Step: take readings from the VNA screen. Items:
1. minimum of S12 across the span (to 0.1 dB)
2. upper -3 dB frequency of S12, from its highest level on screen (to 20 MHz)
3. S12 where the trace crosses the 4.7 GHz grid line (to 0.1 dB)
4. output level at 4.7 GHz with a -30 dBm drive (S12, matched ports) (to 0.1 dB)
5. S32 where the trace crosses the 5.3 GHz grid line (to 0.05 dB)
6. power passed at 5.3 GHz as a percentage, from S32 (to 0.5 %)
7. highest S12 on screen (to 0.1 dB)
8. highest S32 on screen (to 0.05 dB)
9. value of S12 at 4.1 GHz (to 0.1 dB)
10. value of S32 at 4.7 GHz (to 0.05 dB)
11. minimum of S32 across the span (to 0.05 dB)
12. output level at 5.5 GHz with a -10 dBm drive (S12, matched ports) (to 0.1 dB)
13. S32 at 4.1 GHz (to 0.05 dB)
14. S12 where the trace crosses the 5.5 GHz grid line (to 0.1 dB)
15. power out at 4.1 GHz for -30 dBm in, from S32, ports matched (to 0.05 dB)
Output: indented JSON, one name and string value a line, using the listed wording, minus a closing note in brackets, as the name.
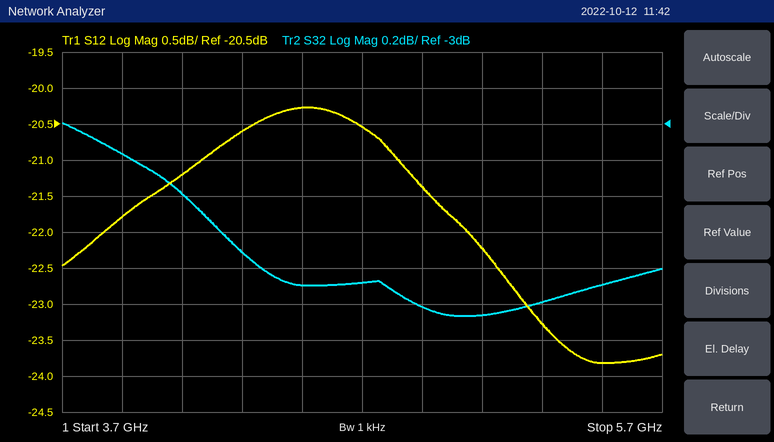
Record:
{
  "minimum of S12 across the span": "-23.8 dB",
  "upper -3 dB frequency of S12, from its highest level on screen": "5.30 GHz",
  "S12 where the trace crosses the 4.7 GHz grid line": "-20.5 dB",
  "output level at 4.7 GHz with a -30 dBm drive (S12, matched ports)": "-50.5 dBm",
  "S32 where the trace crosses the 5.3 GHz grid line": "-4.00 dB",
  "power passed at 5.3 GHz as a percentage, from S32": "40.0 %",
  "highest S12 on screen": "-20.3 dB",
  "highest S32 on screen": "-3.00 dB",
  "value of S12 at 4.1 GHz": "-21.2 dB",
  "value of S32 at 4.7 GHz": "-3.90 dB",
  "minimum of S32 across the span": "-4.05 dB",
  "output level at 5.5 GHz with a -10 dBm drive (S12, matched ports)": "-33.8 dBm",
  "S32 at 4.1 GHz": "-3.40 dB",
  "S12 where the trace crosses the 5.5 GHz grid line": "-23.8 dB",
  "power out at 4.1 GHz for -30 dBm in, from S32, ports matched": "-33.40 dBm"
}
